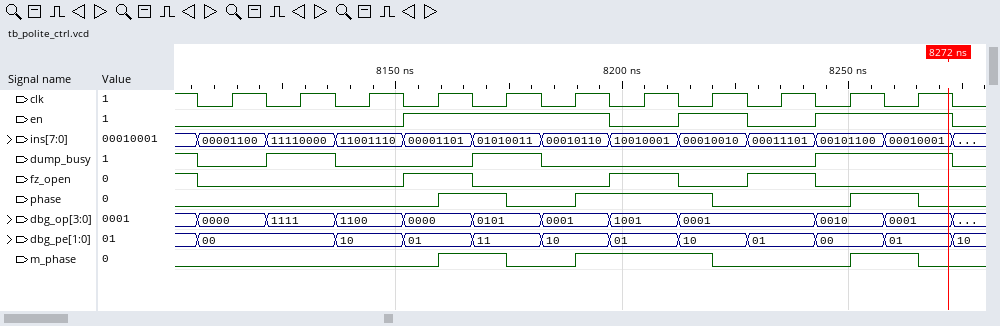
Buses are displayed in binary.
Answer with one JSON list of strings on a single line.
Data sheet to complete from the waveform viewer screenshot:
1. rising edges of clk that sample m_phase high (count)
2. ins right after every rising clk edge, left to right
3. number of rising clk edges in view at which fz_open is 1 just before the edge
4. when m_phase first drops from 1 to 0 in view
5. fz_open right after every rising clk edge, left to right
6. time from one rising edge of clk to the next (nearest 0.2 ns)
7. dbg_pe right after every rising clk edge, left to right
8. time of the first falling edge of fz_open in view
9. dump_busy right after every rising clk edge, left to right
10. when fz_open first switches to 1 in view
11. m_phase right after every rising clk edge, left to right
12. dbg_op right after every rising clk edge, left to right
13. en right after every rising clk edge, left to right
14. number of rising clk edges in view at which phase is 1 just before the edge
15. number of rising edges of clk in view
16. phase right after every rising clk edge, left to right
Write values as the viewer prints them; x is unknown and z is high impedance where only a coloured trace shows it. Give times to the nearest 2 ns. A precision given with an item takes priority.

["4", "00001100, 11110000, 11001110, 00001101, 01010011, 00010110, 10010001, 00010010, 00011101, 00101100, 00010001", "3", "8174 ns", "0 0 0 1 0 0 1 0 1 0 0", "15.2 ns", "00, 00, 10, 01, 11, 10, 01, 10, 01, 00, 01", "8106 ns", "0 1 0 0 1 0 0 0 0 1 1", "8152 ns", "0 0 0 1 0 1 1 0 0 1 0", "0000, 1111, 1100, 0000, 0101, 0001, 1001, 0001, 0001, 0010, 0001", "0 0 0 1 1 1 0 1 0 1 1", "4", "11", "0 0 0 1 0 1 1 0 0 1 0"]
